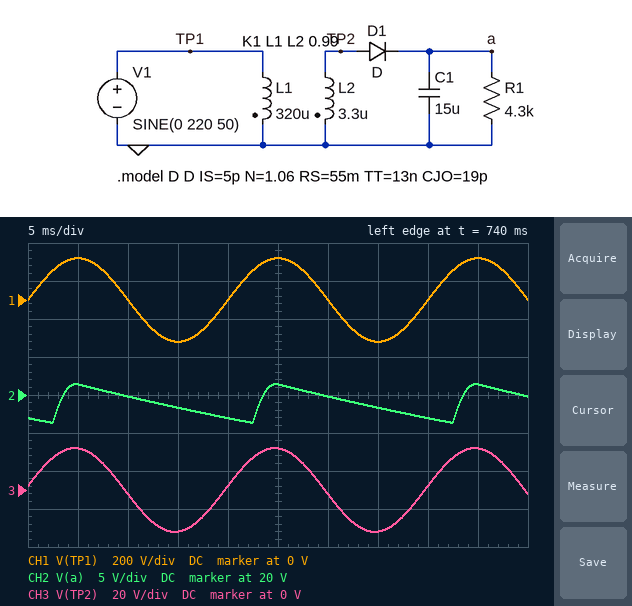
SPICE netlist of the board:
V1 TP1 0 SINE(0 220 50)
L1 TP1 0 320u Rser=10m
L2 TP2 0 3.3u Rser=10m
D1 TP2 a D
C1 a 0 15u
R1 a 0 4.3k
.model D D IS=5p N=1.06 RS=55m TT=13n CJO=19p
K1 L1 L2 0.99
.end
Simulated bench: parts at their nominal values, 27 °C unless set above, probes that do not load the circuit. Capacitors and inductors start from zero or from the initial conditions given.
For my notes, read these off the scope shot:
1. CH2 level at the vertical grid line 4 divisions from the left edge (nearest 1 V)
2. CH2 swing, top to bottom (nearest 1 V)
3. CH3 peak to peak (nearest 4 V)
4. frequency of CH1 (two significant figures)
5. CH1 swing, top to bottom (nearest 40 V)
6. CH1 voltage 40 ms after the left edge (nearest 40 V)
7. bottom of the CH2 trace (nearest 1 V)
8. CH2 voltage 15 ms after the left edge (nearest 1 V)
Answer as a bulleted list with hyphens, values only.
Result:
- 17 V
- 5 V
- 44 V
- 50 Hz
- 440 V
- 0 V
- 16 V
- 18 V
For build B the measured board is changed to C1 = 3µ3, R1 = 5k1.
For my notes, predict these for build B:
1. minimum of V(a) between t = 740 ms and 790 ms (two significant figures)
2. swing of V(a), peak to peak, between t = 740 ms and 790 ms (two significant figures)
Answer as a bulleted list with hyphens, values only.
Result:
- 8.3 V
- 13 V
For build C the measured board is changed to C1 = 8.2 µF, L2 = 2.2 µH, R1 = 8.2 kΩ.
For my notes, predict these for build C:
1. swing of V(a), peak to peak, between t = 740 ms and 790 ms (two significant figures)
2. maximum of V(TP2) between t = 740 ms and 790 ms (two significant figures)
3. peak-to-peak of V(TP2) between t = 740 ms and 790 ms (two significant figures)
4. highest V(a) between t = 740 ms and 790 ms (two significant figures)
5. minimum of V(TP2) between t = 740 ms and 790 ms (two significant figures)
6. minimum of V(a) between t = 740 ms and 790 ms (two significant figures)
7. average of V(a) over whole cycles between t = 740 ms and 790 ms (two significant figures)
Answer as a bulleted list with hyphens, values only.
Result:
- 4.0 V
- 18 V
- 36 V
- 17 V
- -18 V
- 13 V
- 15 V
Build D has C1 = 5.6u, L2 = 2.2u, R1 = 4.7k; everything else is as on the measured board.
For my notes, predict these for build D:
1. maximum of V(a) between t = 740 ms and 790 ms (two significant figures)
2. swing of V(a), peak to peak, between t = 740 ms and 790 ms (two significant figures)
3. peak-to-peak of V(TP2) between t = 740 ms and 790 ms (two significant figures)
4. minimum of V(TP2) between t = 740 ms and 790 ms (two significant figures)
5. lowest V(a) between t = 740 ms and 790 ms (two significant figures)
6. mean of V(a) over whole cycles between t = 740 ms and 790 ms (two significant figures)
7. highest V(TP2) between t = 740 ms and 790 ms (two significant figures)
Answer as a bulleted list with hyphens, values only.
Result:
- 17 V
- 8.1 V
- 36 V
- -18 V
- 9.3 V
- 13 V
- 18 V
